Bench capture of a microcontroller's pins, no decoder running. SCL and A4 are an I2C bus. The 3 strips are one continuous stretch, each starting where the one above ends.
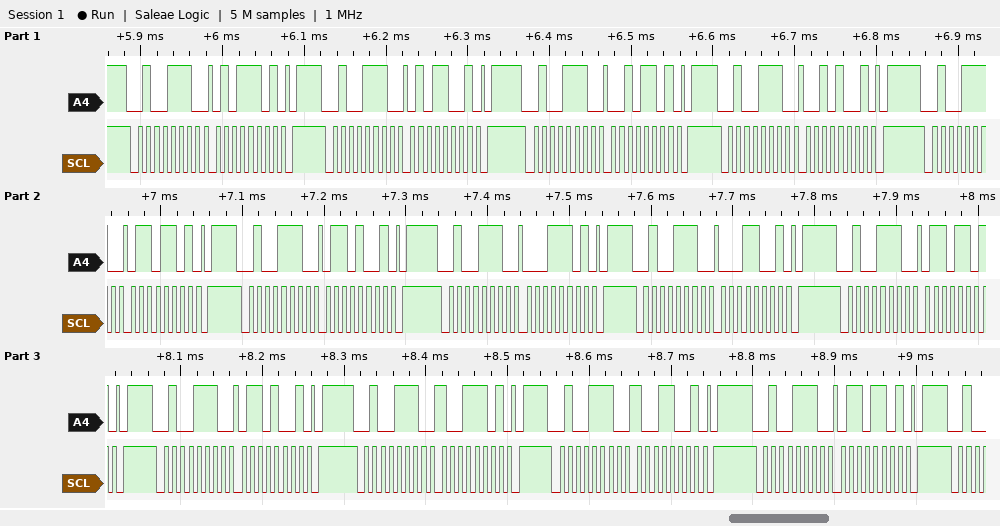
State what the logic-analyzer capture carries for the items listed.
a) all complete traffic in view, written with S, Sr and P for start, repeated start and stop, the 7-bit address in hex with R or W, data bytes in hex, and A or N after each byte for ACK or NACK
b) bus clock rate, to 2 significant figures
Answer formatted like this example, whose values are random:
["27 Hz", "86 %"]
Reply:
["S 27W A 5D A P S 27W A 59 A P S 27W A 2D A P S 27W A 29 A P S 27W A 6D A P S 27W A 69 A P S 27W A 1D A P S 27W A 19 A P S 27W A 6D A P S 27W A 69 A P S 27W A 9D A P S 27W A 99 A P S 27W A 6D A P", "100 kHz"]
